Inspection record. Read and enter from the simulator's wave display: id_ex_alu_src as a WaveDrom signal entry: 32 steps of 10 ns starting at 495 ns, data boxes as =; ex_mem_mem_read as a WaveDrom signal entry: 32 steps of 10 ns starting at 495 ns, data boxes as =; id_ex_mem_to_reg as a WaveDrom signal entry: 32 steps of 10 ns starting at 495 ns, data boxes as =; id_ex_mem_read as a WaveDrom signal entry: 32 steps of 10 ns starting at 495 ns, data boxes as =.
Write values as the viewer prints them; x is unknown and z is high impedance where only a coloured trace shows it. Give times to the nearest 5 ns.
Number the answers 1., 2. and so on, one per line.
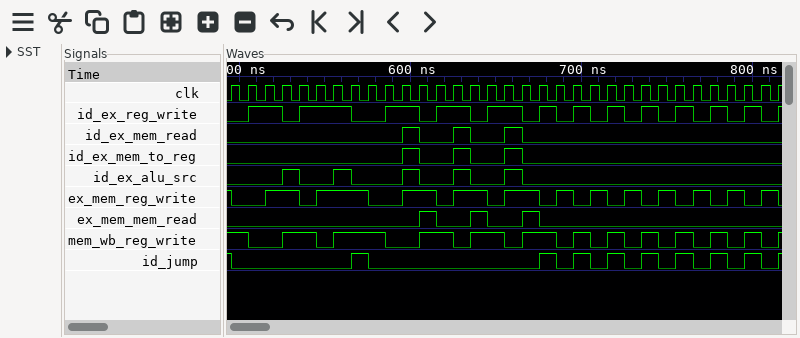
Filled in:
1. {name: 'id_ex_alu_src', wave: '0..10.10..10.10.10..............'}
2. {name: 'ex_mem_mem_read', wave: '0..........10.10.10.............'}
3. {name: 'id_ex_mem_to_reg', wave: '0.........10.10.10..............'}
4. {name: 'id_ex_mem_read', wave: '0.........10.10.10..............'}
